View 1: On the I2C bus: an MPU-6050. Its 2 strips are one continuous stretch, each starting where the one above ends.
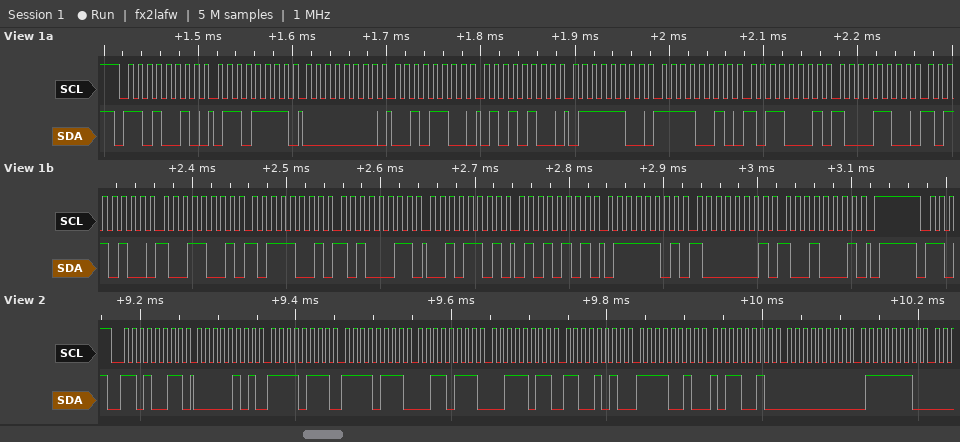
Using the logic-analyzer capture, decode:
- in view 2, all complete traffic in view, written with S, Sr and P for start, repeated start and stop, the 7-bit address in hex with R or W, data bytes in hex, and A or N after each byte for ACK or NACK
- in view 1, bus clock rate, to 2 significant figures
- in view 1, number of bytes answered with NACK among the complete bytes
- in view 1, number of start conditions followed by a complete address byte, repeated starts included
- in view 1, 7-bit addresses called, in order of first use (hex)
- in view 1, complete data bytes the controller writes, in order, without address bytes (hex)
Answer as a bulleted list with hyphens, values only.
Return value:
- S 69R A 05 A F7 A F7 A 37 A 3B A CA A F2 A B2 A 00 A 7E A
- 100 kHz
- 0
- 1
- 0x69
- 6F 00 2C 54 7C F2 B1 8C B4 99 B9 A3 2D 55 7D 81 91
